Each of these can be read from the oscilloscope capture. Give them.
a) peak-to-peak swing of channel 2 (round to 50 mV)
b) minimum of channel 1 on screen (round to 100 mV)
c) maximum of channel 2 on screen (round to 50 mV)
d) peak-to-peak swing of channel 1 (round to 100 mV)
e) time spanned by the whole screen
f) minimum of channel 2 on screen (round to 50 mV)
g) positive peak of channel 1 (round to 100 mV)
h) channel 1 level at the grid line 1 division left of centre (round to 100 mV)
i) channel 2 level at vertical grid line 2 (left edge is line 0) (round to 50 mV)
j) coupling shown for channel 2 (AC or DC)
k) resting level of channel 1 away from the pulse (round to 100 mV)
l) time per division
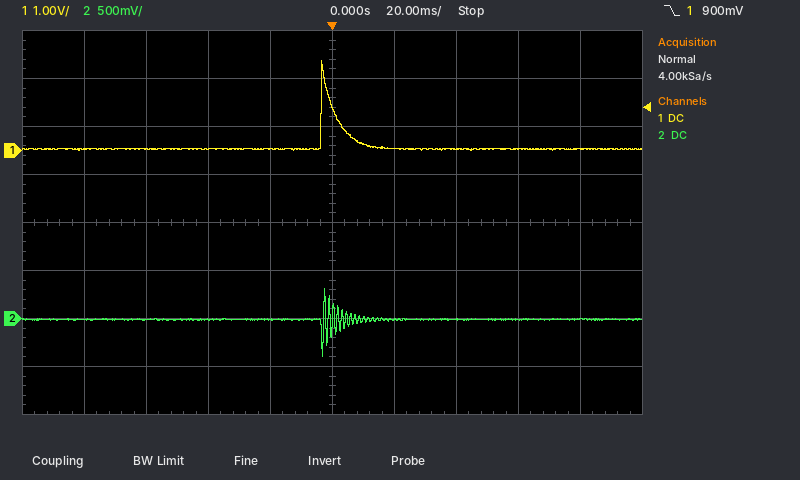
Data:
700 mV
0.0 V
300 mV
1.9 V
200 ms
-400 mV
1.9 V
0.0 V
0 mV
DC
0.0 V
20 ms
